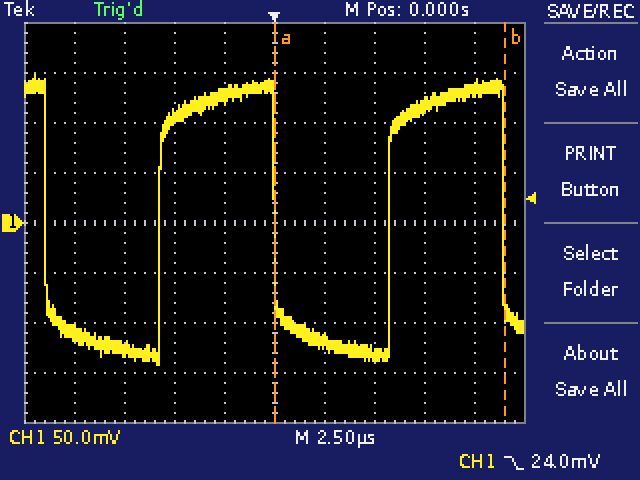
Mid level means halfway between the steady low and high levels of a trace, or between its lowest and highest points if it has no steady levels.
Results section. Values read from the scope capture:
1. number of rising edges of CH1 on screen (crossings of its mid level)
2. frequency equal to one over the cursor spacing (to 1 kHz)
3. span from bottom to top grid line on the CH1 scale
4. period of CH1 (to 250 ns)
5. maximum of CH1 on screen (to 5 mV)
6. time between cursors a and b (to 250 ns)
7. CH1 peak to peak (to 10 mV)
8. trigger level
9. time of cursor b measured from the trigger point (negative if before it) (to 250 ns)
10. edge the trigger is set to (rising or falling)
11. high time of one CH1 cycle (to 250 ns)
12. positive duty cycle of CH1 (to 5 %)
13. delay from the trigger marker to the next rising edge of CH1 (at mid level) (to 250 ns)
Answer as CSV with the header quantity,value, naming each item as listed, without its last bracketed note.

quantity,value
number of rising edges of CH1 on screen,2
frequency equal to one over the cursor spacing,87 kHz
span from bottom to top grid line on the CH1 scale,400 mV
period of CH1,11.50 µs
maximum of CH1 on screen,150 mV
time between cursors a and b,11.50 µs
CH1 peak to peak,290 mV
trigger level,24.0 mV
time of cursor b measured from the trigger point (negative if before it),+11.50 µs
edge the trigger is set to,falling
high time of one CH1 cycle,5.75 µs
positive duty cycle of CH1,50 %
delay from the trigger marker to the next rising edge of CH1 (at mid level),5.75 µs
